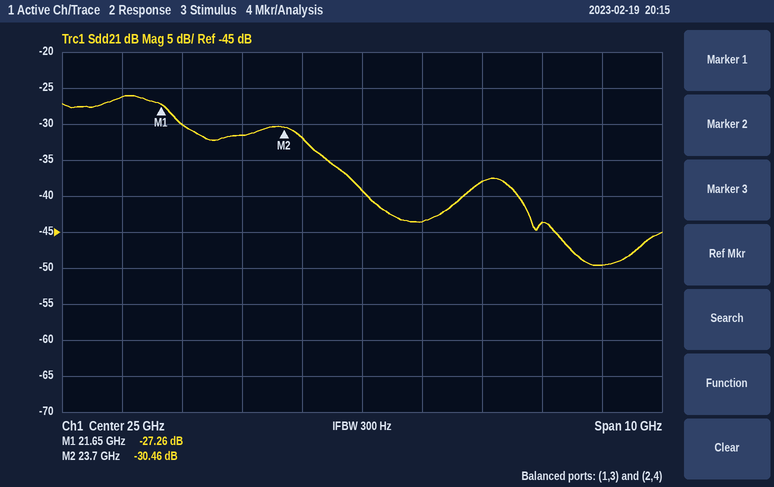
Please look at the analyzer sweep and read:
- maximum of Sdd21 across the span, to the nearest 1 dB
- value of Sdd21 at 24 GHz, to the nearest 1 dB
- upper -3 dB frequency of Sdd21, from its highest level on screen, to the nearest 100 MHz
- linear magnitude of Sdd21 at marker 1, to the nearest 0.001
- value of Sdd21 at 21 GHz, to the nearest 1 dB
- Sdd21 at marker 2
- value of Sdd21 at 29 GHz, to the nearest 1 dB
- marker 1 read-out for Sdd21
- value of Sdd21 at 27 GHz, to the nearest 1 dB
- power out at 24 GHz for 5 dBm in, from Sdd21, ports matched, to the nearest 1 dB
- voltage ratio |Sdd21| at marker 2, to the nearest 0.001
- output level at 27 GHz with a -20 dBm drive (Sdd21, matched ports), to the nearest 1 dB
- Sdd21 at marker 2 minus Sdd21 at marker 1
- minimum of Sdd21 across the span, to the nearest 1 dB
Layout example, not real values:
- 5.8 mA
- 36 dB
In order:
- -26 dB
- -32 dB
- 21.9 GHz
- 0.043
- -26 dB
- -30.46 dB
- -50 dB
- -27.26 dB
- -38 dB
- -27 dBm
- 0.030
- -58 dBm
- -3.20 dB
- -50 dB
